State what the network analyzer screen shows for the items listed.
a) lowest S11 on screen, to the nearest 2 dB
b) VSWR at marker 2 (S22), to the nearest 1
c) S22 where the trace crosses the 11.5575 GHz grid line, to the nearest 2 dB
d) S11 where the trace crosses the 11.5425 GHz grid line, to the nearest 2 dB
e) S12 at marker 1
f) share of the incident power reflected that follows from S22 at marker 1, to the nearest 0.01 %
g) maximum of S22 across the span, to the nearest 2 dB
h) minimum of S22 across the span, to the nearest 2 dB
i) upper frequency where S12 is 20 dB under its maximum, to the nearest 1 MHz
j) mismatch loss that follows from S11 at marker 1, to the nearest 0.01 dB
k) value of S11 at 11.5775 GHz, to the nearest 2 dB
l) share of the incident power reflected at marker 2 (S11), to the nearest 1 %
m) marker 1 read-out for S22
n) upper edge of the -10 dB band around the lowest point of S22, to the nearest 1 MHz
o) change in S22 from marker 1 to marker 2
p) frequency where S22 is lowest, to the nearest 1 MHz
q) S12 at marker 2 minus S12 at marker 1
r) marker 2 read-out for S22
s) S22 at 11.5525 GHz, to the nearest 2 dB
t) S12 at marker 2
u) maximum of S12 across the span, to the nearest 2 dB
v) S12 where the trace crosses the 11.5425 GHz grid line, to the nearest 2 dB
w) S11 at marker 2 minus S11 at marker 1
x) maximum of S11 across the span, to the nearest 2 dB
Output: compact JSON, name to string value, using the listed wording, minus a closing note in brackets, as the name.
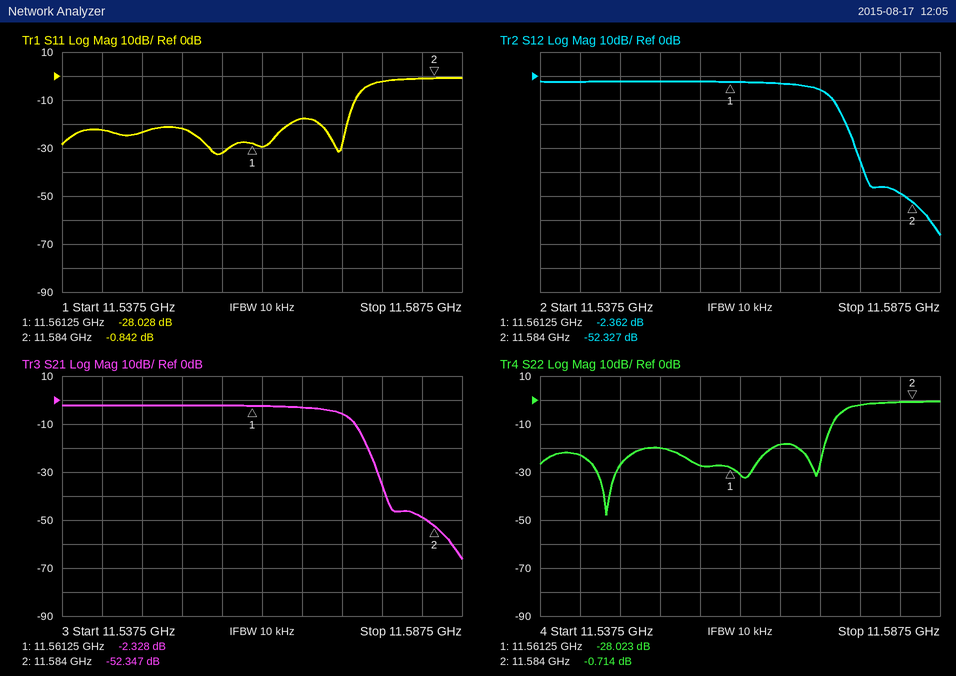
{"lowest S11 on screen, to the nearest 2 dB": "-32 dB", "VSWR at marker 2 (S22), to the nearest 1": "24", "S22 where the trace crosses the 11.5575 GHz grid line, to the nearest 2 dB": "-28 dB", "S11 where the trace crosses the 11.5425 GHz grid line, to the nearest 2 dB": "-22 dB", "S12 at marker 1": "-2.362 dB", "share of the incident power reflected that follows from S22 at marker 1, to the nearest 0.01 %": "0.16 %", "maximum of S22 across the span, to the nearest 2 dB": "0 dB", "minimum of S22 across the span, to the nearest 2 dB": "-48 dB", "upper frequency where S12 is 20 dB under its maximum, to the nearest 1 MHz": "11.576 GHz", "mismatch loss that follows from S11 at marker 1, to the nearest 0.01 dB": "0.01 dB", "value of S11 at 11.5775 GHz, to the nearest 2 dB": "-2 dB", "share of the incident power reflected at marker 2 (S11), to the nearest 1 %": "82 %", "marker 1 read-out for S22": "-28.023 dB", "upper edge of the -10 dB band around the lowest point of S22, to the nearest 1 MHz": "11.574 GHz", "change in S22 from marker 1 to marker 2": "27.309 dB", "frequency where S22 is lowest, to the nearest 1 MHz": "11.546 GHz", "S12 at marker 2 minus S12 at marker 1": "-49.965 dB", "marker 2 read-out for S22": "-0.714 dB", "S22 at 11.5525 GHz, to the nearest 2 dB": "-20 dB", "S12 at marker 2": "-52.327 dB", "maximum of S12 across the span, to the nearest 2 dB": "-2 dB", "S12 where the trace crosses the 11.5425 GHz grid line, to the nearest 2 dB": "-2 dB", "S11 at marker 2 minus S11 at marker 1": "27.186 dB", "maximum of S11 across the span, to the nearest 2 dB": "0 dB"}
